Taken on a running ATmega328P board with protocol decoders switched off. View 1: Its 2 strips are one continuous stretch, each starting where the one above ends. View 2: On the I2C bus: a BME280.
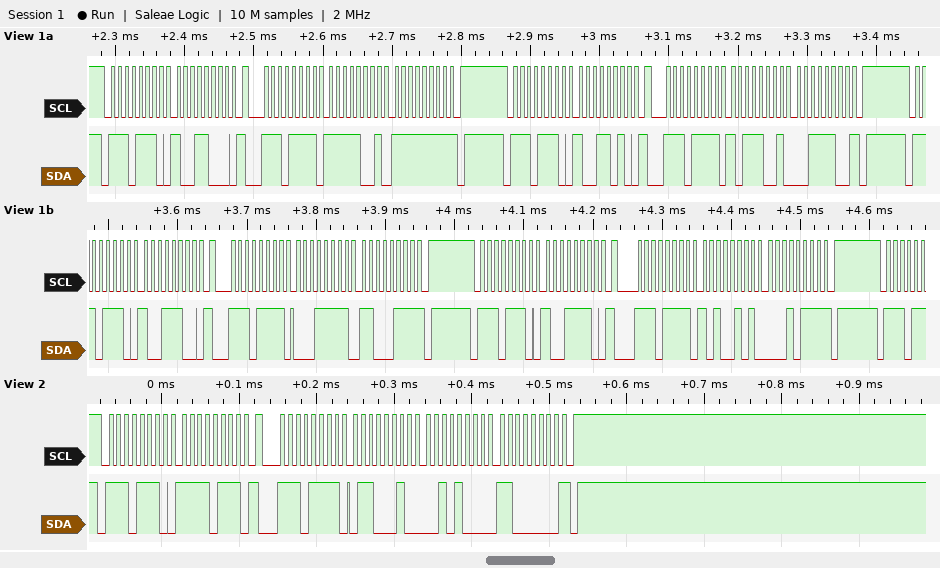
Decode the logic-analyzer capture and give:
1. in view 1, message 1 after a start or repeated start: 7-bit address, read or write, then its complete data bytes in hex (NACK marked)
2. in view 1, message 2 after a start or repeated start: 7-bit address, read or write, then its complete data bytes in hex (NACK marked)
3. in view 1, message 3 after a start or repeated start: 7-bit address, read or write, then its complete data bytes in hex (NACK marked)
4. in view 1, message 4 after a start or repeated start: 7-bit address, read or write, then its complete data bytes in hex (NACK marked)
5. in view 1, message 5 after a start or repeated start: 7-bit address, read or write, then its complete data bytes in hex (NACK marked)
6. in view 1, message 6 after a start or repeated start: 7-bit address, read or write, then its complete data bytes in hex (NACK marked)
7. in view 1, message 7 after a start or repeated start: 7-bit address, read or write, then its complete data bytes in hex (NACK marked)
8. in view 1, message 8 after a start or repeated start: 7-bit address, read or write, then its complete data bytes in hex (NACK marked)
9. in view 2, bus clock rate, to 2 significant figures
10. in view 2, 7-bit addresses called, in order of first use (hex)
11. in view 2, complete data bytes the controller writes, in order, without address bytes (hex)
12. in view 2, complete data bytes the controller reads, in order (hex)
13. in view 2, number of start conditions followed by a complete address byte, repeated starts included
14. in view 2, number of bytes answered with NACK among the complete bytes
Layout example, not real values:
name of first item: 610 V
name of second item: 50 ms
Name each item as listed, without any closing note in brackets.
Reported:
in view 1, message 1 after a start or repeated start: 7-bit address, read or write, then its complete data bytes in hex: 0x77 write: 98
in view 1, message 2 after a start or repeated start: 7-bit address, read or write, then its complete data bytes in hex: 0x77 read: F9 FF NACK
in view 1, message 3 after a start or repeated start: 7-bit address, read or write, then its complete data bytes in hex: 0x77 write: 9A
in view 1, message 4 after a start or repeated start: 7-bit address, read or write, then its complete data bytes in hex: 0x77 read: B9 3C NACK
in view 1, message 5 after a start or repeated start: 7-bit address, read or write, then its complete data bytes in hex: 0x77 write: 9C
in view 1, message 6 after a start or repeated start: 7-bit address, read or write, then its complete data bytes in hex: 0x77 read: 1F C7 NACK
in view 1, message 7 after a start or repeated start: 7-bit address, read or write, then its complete data bytes in hex: 0x77 write: 9E
in view 1, message 8 after a start or repeated start: 7-bit address, read or write, then its complete data bytes in hex: 0x77 read: A5 17 NACK
in view 2, bus clock rate, to 2 significant figures: 100 kHz
in view 2, 7-bit addresses called, in order of first use: 0x77
in view 2, complete data bytes the controller writes, in order, without address bytes: F7
in view 2, complete data bytes the controller reads, in order: 62 28 C0
in view 2, number of start conditions followed by a complete address byte, repeated starts included: 2
in view 2, number of bytes answered with NACK among the complete bytes: 1
